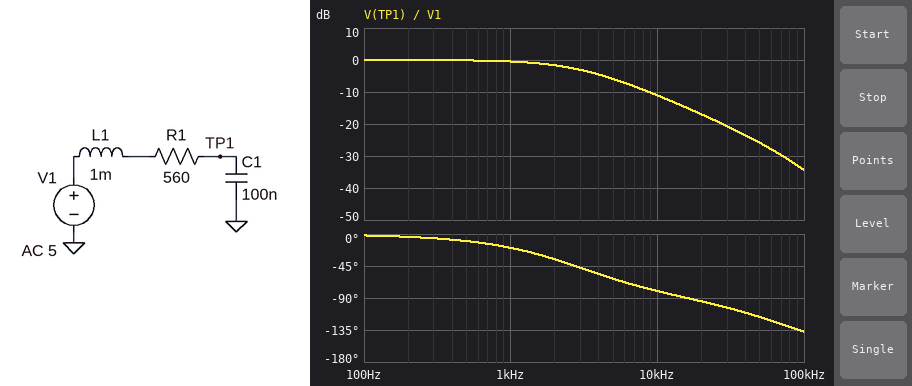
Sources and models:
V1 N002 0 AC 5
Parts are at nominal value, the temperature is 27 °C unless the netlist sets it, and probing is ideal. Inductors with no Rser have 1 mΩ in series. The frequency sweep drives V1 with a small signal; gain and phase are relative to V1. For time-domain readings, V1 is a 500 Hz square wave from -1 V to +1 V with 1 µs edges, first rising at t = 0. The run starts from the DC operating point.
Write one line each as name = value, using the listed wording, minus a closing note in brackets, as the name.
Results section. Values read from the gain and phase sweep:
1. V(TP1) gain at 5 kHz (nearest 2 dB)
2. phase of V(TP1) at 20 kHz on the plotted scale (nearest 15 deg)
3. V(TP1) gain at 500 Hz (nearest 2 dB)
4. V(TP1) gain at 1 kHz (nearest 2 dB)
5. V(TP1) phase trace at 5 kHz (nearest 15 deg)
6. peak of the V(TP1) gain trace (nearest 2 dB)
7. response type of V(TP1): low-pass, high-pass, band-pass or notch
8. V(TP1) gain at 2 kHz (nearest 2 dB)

V(TP1) gain at 5 kHz = -6 dB
phase of V(TP1) at 20 kHz on the plotted scale = -90 deg
V(TP1) gain at 500 Hz = 0 dB
V(TP1) gain at 1 kHz = 0 dB
V(TP1) phase trace at 5 kHz = -60 deg
peak of the V(TP1) gain trace = 0 dB
response type of V(TP1): low-pass, high-pass, band-pass or notch = low-pass
V(TP1) gain at 2 kHz = -2 dB
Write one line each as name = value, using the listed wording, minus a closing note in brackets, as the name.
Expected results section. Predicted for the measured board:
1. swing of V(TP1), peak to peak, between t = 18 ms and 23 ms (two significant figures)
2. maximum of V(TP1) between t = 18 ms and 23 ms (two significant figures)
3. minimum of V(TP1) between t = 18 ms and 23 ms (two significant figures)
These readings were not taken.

swing of V(TP1), peak to peak, between t = 18 ms and 23 ms = 2.0 V
maximum of V(TP1) between t = 18 ms and 23 ms = 1.0 V
minimum of V(TP1) between t = 18 ms and 23 ms = -1.0 V
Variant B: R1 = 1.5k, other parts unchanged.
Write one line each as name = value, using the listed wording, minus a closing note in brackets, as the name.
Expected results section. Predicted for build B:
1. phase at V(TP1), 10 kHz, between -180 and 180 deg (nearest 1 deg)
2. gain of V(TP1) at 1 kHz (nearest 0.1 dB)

phase at V(TP1), 10 kHz, between -180 and 180 deg = -86 deg
gain of V(TP1) at 1 kHz = -2.7 dB
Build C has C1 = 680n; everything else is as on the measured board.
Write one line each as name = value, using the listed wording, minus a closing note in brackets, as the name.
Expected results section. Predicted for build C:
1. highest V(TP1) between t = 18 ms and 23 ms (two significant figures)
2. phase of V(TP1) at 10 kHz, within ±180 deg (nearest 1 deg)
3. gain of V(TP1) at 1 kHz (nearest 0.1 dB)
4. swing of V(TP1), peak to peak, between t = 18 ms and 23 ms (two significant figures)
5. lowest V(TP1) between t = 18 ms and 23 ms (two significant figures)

highest V(TP1) between t = 18 ms and 23 ms = 870 mV
phase of V(TP1) at 10 kHz, within ±180 deg = -94 deg
gain of V(TP1) at 1 kHz = -8.2 dB
swing of V(TP1), peak to peak, between t = 18 ms and 23 ms = 1.7 V
lowest V(TP1) between t = 18 ms and 23 ms = -870 mV
